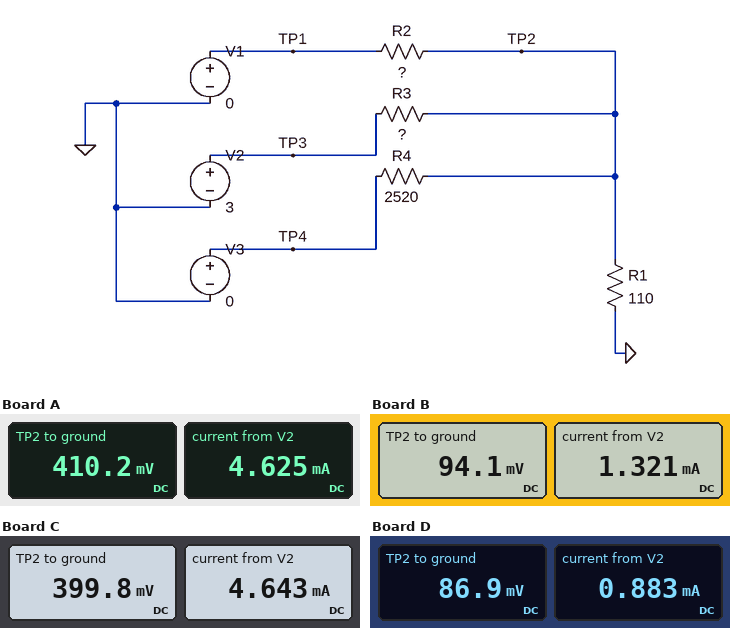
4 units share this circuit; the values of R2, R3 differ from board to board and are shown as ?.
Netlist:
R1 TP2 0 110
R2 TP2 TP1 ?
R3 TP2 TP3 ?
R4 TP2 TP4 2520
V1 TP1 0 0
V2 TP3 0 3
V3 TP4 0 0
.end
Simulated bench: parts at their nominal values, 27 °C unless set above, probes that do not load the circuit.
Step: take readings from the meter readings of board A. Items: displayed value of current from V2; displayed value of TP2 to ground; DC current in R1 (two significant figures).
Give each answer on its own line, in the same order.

4.625 mA
410.2 mV
3.7 mA
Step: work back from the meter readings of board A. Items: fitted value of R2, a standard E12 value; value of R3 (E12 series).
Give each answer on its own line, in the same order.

560 Ω
560 Ω
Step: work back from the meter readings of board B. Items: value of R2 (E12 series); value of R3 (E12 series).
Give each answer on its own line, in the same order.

220 Ω
2.2 kΩ
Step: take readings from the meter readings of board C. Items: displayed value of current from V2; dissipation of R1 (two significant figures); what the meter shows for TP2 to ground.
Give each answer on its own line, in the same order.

4.643 mA
1.5 mW
399.8 mV
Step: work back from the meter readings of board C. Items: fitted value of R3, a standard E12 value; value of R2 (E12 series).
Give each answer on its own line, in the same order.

560 Ω
470 Ω
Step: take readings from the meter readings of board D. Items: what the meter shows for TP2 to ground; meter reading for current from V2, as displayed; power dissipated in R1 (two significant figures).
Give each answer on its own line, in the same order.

86.9 mV
0.883 mA
69 µW
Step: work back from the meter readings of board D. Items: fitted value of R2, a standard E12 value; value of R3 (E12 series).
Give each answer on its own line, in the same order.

1.5 kΩ
3.3 kΩ
